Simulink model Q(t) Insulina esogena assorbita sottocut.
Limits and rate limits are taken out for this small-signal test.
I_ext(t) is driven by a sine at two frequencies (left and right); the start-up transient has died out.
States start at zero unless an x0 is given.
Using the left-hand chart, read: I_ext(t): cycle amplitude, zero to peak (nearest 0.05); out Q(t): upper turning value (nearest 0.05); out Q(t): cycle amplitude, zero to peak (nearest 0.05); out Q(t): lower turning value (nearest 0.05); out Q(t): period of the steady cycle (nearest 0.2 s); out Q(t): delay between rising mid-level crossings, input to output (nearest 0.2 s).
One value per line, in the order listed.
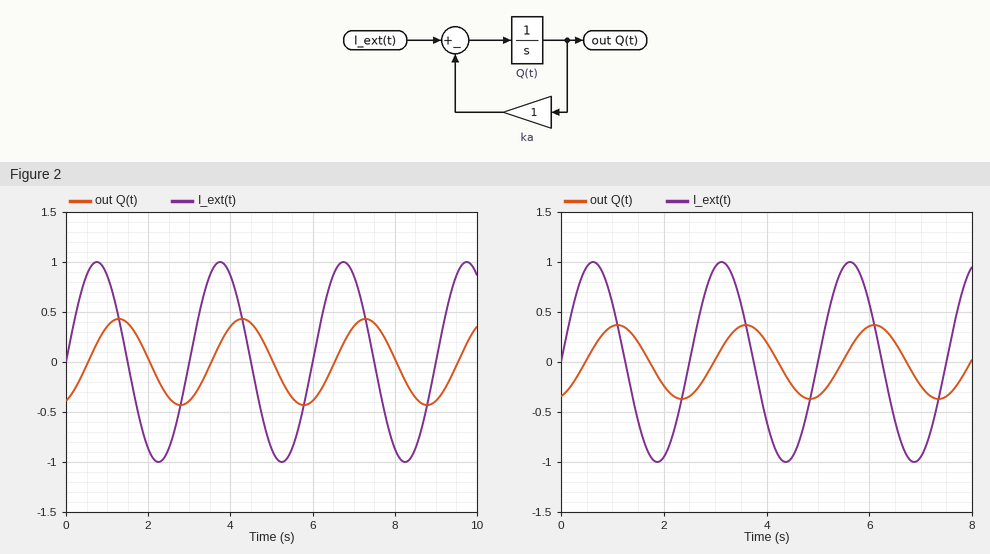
1.00
0.45
0.45
-0.45
3.0 s
0.6 s
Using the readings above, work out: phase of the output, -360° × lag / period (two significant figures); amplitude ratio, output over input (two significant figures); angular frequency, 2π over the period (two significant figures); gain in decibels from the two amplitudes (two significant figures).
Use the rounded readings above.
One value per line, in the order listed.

-72°
0.45
2.1 rad/s
-6.9 dB
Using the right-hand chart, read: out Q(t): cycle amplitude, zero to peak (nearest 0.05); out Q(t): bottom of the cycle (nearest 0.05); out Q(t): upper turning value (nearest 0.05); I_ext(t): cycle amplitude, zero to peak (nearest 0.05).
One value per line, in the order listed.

0.35
-0.35
0.35
1.00
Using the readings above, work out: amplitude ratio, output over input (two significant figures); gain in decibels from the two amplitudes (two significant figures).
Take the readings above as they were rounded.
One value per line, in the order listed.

0.35
-9.1 dB
